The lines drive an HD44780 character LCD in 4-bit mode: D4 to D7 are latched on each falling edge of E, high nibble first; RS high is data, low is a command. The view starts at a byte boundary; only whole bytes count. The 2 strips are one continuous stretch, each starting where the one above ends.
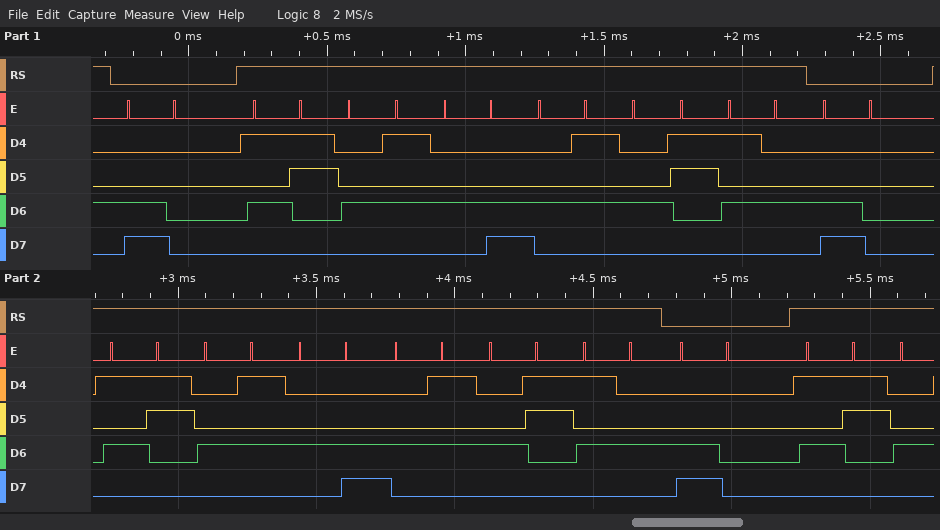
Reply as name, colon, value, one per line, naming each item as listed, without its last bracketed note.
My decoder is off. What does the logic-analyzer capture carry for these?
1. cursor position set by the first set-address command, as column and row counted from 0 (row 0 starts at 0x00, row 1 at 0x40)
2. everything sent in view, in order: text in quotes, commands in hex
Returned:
cursor position set by the first set-address command, as column and row counted from 0: column 0, row 1
everything sent in view, in order: text in quotes, commands in hex: 0xC0 "SELECT" 0xC0 "SELECT" 0xC0 "S"
